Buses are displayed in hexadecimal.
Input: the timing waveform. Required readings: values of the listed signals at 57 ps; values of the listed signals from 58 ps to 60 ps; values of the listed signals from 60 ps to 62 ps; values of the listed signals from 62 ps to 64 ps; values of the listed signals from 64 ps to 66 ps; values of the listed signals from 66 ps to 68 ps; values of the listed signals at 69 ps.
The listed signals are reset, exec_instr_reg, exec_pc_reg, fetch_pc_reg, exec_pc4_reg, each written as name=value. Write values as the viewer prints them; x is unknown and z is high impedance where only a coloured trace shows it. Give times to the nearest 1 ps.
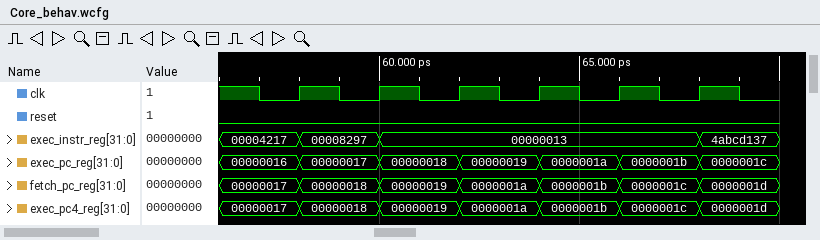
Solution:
reset=0, exec_instr_reg=00004217, exec_pc_reg=00000016, fetch_pc_reg=00000017, exec_pc4_reg=00000017
reset=0, exec_instr_reg=00008297, exec_pc_reg=00000017, fetch_pc_reg=00000018, exec_pc4_reg=00000018
reset=0, exec_instr_reg=00000013, exec_pc_reg=00000018, fetch_pc_reg=00000019, exec_pc4_reg=00000019
reset=0, exec_instr_reg=00000013, exec_pc_reg=00000019, fetch_pc_reg=0000001a, exec_pc4_reg=0000001a
reset=0, exec_instr_reg=00000013, exec_pc_reg=0000001a, fetch_pc_reg=0000001b, exec_pc4_reg=0000001b
reset=0, exec_instr_reg=00000013, exec_pc_reg=0000001b, fetch_pc_reg=0000001c, exec_pc4_reg=0000001c
reset=0, exec_instr_reg=4abcd137, exec_pc_reg=0000001c, fetch_pc_reg=0000001d, exec_pc4_reg=0000001d
